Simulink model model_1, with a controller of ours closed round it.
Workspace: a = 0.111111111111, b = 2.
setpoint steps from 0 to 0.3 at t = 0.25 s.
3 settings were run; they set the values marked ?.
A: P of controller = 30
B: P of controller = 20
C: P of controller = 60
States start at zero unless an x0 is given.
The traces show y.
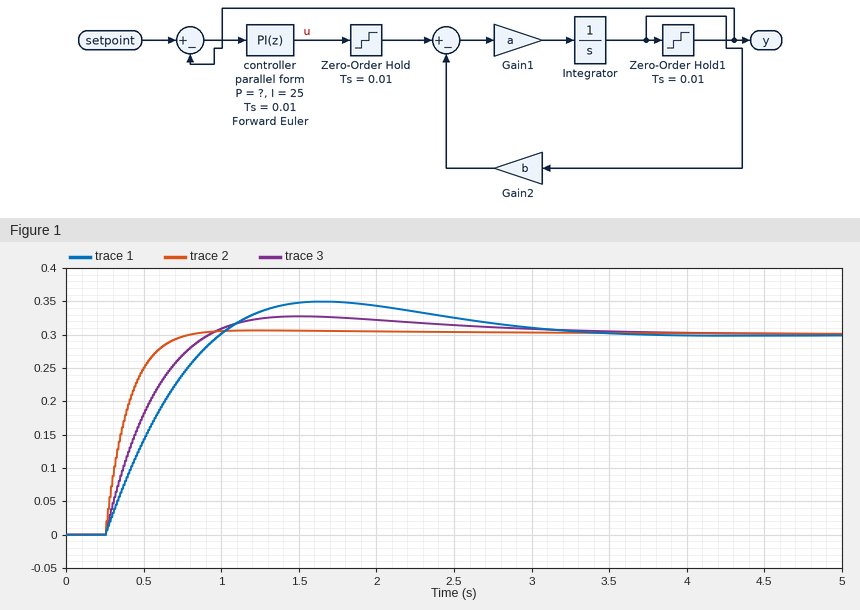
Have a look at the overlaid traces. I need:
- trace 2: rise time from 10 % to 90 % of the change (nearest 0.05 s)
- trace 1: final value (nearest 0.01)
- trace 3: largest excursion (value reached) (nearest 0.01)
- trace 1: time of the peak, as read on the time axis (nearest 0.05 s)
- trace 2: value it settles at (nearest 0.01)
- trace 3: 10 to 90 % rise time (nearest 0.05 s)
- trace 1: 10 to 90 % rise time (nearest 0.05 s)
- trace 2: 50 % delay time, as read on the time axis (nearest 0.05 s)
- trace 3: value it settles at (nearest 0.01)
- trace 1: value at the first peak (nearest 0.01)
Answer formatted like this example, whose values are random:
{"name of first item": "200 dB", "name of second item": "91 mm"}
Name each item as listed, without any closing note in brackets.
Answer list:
{"trace 2: rise time from 10 % to 90 % of the change": "0.30 s", "trace 1: final value": "0.30", "trace 3: largest excursion (value reached)": "0.33", "trace 1: time of the peak, as read on the time axis": "1.65 s", "trace 2: value it settles at": "0.30", "trace 3: 10 to 90 % rise time": "0.45 s", "trace 1: 10 to 90 % rise time": "0.55 s", "trace 2: 50 % delay time, as read on the time axis": "0.35 s", "trace 3: value it settles at": "0.30", "trace 1: value at the first peak": "0.35"}
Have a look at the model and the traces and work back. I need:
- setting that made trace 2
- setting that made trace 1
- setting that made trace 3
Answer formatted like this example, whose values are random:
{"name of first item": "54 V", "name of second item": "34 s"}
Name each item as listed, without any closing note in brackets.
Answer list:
{"setting that made trace 2": "C", "setting that made trace 1": "B", "setting that made trace 3": "A"}
